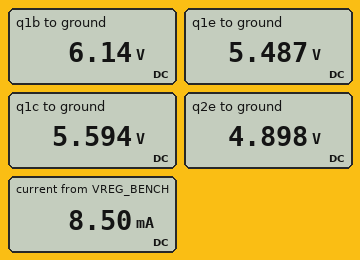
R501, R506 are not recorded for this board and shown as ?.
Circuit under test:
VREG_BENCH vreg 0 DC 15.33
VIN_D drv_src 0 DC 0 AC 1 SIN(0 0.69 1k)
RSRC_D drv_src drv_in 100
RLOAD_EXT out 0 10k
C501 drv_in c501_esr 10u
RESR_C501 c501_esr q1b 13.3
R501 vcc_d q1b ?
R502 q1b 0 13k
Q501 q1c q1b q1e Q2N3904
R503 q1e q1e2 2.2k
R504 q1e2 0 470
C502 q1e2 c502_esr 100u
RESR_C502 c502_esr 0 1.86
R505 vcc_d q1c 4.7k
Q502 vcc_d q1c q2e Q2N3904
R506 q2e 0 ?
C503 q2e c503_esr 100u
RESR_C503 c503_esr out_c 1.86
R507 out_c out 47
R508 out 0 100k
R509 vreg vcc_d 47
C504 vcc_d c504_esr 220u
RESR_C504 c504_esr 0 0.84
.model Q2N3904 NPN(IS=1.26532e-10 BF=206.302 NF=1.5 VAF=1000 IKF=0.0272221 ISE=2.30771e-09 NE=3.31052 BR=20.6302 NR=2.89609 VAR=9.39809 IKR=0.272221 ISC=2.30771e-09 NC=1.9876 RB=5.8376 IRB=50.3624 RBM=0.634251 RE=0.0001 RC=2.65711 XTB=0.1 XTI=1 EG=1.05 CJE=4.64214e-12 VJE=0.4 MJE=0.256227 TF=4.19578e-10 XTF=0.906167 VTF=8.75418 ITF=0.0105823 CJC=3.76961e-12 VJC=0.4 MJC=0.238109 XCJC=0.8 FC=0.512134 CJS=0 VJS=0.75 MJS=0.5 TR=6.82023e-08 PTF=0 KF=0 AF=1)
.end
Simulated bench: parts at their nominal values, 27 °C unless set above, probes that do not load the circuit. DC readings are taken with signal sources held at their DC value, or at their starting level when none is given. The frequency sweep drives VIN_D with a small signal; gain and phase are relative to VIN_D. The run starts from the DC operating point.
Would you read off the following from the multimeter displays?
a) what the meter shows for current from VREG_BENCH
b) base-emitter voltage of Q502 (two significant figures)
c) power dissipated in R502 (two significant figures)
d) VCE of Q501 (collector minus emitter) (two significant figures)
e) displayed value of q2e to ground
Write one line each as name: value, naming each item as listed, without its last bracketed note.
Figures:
what the meter shows for current from VREG_BENCH: 8.50 mA
base-emitter voltage of Q502: 700 mV
power dissipated in R502: 2.9 mW
VCE of Q501 (collector minus emitter): 110 mV
displayed value of q2e to ground: 4.898 V
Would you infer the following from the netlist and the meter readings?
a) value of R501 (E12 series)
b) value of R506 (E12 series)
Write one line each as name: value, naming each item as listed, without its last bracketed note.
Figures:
value of R501: 15 kΩ
value of R506: 820 Ω
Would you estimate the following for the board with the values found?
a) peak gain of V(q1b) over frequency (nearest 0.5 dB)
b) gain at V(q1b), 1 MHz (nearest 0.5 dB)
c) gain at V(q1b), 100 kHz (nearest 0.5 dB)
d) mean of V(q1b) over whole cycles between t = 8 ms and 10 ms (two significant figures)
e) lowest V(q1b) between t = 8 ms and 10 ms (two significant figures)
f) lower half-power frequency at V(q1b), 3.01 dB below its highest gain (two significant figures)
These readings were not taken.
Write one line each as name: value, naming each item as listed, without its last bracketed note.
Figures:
peak gain of V(q1b) over frequency: -0.5 dB
gain at V(q1b), 1 MHz: -0.5 dB
gain at V(q1b), 100 kHz: -0.5 dB
mean of V(q1b) over whole cycles between t = 8 ms and 10 ms: 6.1 V
lowest V(q1b) between t = 8 ms and 10 ms: 5.4 V
lower half-power frequency at V(q1b), 3.01 dB below its highest gain: 11 Hz
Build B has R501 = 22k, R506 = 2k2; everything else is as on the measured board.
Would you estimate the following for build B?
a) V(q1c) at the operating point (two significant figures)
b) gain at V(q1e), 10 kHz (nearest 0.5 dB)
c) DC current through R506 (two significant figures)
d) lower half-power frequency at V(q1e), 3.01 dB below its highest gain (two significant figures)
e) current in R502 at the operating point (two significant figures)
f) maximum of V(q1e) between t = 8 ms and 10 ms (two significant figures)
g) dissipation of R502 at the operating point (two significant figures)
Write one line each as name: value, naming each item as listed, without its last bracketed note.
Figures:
V(q1c) at the operating point: 6.5 V
gain at V(q1e), 10 kHz: 0 dB
DC current through R506: 2.7 mA
lower half-power frequency at V(q1e), 3.01 dB below its highest gain: 1.9 Hz
current in R502 at the operating point: 420 µA
maximum of V(q1e) between t = 8 ms and 10 ms: 5.5 V
dissipation of R502 at the operating point: 2.3 mW
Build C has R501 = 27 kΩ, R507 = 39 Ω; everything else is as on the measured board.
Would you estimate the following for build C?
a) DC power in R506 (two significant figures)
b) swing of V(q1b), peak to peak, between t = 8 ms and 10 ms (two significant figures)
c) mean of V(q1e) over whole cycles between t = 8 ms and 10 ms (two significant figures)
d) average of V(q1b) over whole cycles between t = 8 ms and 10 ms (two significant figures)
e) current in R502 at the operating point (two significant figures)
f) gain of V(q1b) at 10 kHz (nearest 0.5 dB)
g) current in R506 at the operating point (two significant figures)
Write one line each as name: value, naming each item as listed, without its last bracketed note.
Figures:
DC power in R506: 55 mW
swing of V(q1b), peak to peak, between t = 8 ms and 10 ms: 1.4 V
mean of V(q1e) over whole cycles between t = 8 ms and 10 ms: 4.1 V
average of V(q1b) over whole cycles between t = 8 ms and 10 ms: 4.7 V
current in R502 at the operating point: 360 µA
gain of V(q1b) at 10 kHz: 0 dB
current in R506 at the operating point: 8.2 mA
